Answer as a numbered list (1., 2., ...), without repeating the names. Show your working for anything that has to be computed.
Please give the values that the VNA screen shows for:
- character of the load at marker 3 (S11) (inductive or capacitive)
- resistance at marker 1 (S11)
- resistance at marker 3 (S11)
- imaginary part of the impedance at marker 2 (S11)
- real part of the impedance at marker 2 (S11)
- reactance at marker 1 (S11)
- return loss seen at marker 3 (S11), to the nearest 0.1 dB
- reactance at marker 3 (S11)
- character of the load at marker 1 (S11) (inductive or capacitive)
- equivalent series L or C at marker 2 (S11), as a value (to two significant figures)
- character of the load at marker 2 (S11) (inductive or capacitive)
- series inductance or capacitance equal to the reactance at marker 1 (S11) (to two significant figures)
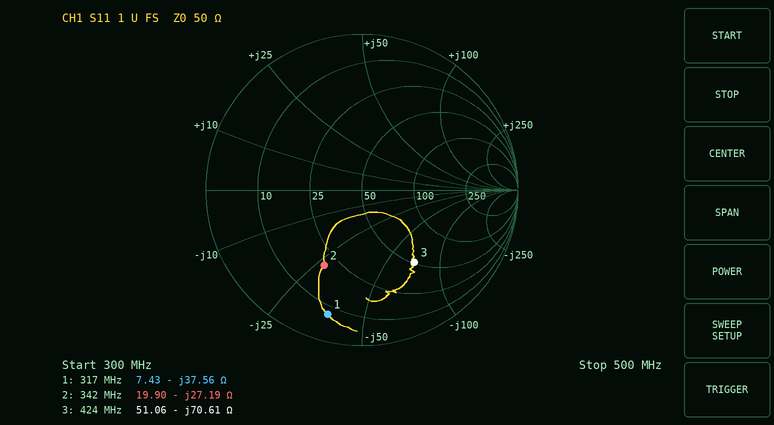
1. capacitive
2. 7.43 Ω
3. 51.06 Ω
4. -27.19 Ω
5. 19.90 Ω
6. -37.56 Ω
7. 4.8 dB
8. -70.61 Ω
9. capacitive
10. C = 1/(2π × 342 MHz × 27.19 Ω) ≈ 17 pF
11. capacitive
12. C = 1/(2π × 317 MHz × 37.56 Ω) ≈ 13 pF
